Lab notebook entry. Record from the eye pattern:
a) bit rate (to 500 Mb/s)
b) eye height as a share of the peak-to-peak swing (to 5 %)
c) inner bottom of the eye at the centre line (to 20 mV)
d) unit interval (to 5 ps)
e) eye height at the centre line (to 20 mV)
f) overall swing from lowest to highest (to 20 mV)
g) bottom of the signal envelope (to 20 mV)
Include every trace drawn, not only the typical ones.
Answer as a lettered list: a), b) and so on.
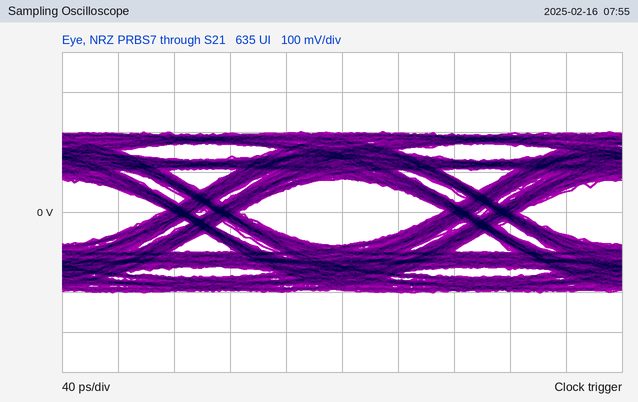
a) 5.0 Gb/s
b) 40 %
c) -80 mV
d) 200 ps
e) 160 mV
f) 400 mV
g) -200 mV
